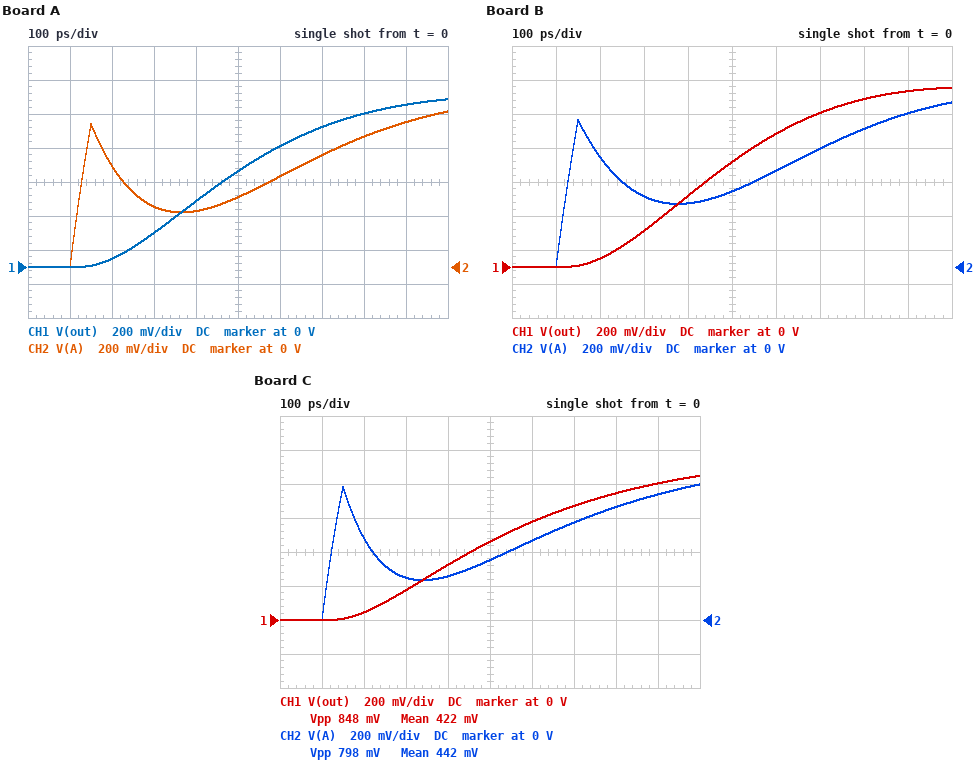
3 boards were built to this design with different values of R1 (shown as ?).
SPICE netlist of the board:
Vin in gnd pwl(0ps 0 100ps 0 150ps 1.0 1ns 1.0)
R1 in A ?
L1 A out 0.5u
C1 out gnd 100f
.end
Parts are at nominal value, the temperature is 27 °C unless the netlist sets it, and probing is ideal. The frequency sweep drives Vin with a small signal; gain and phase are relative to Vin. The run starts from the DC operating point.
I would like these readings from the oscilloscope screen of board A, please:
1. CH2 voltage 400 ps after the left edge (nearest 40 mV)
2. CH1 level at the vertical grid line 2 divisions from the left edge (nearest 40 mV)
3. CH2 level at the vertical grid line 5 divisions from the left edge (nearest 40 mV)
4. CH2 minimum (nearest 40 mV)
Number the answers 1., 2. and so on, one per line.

1. 320 mV
2. 40 mV
3. 400 mV
4. 0 V
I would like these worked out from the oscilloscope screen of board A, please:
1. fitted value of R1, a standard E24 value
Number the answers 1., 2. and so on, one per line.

1. 3.6 kΩ
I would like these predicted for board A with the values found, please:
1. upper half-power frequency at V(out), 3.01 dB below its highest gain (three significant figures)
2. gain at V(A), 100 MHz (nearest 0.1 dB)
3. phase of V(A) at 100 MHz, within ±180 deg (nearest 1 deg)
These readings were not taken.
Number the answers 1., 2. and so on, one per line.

1. 615 MHz
2. -0.2 dB
3. -13 deg
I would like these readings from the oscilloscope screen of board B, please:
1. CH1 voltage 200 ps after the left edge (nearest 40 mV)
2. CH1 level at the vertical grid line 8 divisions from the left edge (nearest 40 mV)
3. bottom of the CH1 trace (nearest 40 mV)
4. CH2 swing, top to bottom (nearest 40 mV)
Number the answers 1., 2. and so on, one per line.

1. 40 mV
2. 1.00 V
3. 0 V
4. 960 mV
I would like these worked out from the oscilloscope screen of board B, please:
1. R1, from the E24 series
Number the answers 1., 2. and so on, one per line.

1. 3 kΩ
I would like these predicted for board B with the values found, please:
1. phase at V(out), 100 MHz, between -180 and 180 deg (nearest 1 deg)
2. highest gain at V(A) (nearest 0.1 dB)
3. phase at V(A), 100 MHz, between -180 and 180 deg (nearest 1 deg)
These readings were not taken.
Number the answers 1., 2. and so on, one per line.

1. -11 deg
2. 0 dB
3. -11 deg
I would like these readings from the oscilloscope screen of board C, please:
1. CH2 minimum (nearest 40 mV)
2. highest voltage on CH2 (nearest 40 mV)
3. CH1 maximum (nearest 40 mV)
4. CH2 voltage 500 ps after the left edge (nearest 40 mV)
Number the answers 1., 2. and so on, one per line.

1. 0 V
2. 800 mV
3. 840 mV
4. 360 mV
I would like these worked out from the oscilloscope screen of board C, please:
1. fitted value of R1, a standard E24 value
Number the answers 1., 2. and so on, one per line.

1. 5.1 kΩ
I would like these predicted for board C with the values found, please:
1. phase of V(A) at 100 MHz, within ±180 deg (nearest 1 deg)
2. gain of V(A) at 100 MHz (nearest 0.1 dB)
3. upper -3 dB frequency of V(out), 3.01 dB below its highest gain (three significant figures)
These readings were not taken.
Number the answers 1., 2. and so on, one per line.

1. -18 deg
2. -0.4 dB
3. 381 MHz
